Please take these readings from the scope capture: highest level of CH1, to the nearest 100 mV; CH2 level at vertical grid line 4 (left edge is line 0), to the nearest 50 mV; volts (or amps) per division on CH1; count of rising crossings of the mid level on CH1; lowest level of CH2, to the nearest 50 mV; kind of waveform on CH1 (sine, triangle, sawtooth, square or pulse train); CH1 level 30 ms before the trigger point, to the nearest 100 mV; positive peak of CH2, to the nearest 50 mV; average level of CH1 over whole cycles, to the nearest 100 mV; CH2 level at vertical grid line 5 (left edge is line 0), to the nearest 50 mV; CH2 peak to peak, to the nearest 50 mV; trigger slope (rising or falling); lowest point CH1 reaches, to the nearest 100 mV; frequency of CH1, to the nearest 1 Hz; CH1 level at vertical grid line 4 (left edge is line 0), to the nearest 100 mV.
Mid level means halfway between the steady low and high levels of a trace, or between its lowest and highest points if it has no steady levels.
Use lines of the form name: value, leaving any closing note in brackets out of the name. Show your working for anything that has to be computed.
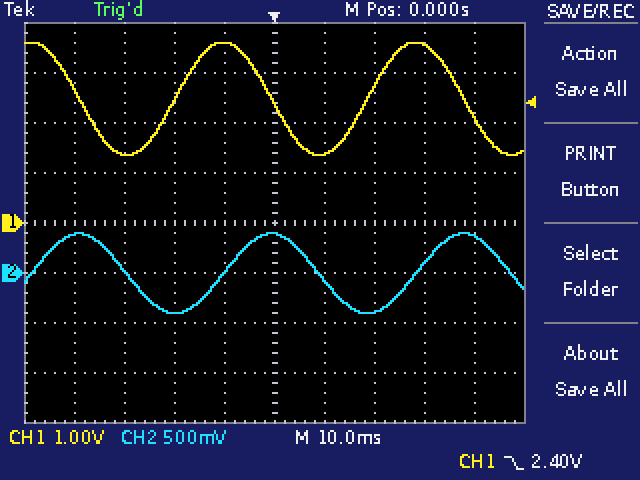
highest level of CH1, to the nearest 100 mV: 3.6 V
CH2 level at vertical grid line 4 (left edge is line 0), to the nearest 50 mV: 0 mV
volts (or amps) per division on CH1: 1 V
count of rising crossings of the mid level on CH1: 2
lowest level of CH2, to the nearest 50 mV: -400 mV
kind of waveform on CH1: sine
CH1 level 30 ms before the trigger point, to the nearest 100 mV: 1.4 V
positive peak of CH2, to the nearest 50 mV: 400 mV
average level of CH1 over whole cycles, to the nearest 100 mV: (3.6 V + (1.4 V)) / 2 ≈ 2.5 V
CH2 level at vertical grid line 5 (left edge is line 0), to the nearest 50 mV: 400 mV
CH2 peak to peak, to the nearest 50 mV: 400 mV − (-400 mV) = 800 mV
trigger slope: falling
lowest point CH1 reaches, to the nearest 100 mV: 1.4 V
frequency of CH1, to the nearest 1 Hz: 26 Hz
CH1 level at vertical grid line 4 (left edge is line 0), to the nearest 100 mV: 3.6 V
